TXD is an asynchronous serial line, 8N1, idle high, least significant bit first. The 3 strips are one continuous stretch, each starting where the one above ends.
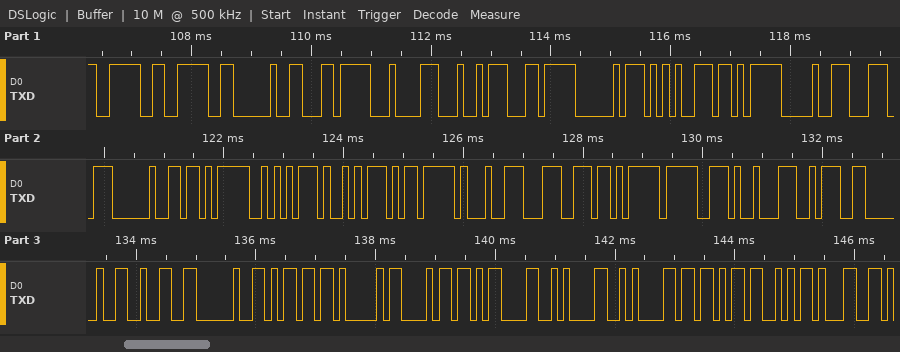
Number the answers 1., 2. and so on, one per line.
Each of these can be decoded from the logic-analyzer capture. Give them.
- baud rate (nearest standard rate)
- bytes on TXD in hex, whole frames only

1. 9600 baud
2. 3E 3E 20 EC 84 A4 EC A0 95 EB 90 9C 20 EB AA A9 ED 91 9C EB 9F 89 3A 20 32 20 6D 41 68 0D 0A 0A 5B 53 31
